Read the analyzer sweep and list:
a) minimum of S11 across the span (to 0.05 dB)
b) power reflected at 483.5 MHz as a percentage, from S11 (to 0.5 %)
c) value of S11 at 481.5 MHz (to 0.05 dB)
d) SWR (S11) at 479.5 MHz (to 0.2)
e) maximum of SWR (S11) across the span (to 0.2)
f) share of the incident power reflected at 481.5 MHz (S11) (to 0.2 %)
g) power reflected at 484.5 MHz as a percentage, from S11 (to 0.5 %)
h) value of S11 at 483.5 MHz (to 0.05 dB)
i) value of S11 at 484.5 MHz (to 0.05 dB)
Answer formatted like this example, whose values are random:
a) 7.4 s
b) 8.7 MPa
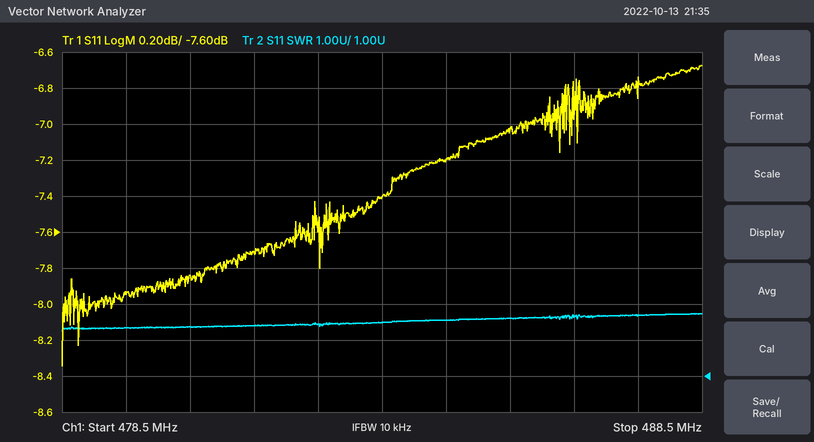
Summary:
a) -8.35 dB
b) 18.0 %
c) -7.70 dB
d) 2.4
e) 2.8
f) 17.0 %
g) 19.0 %
h) -7.40 dB
i) -7.20 dB
